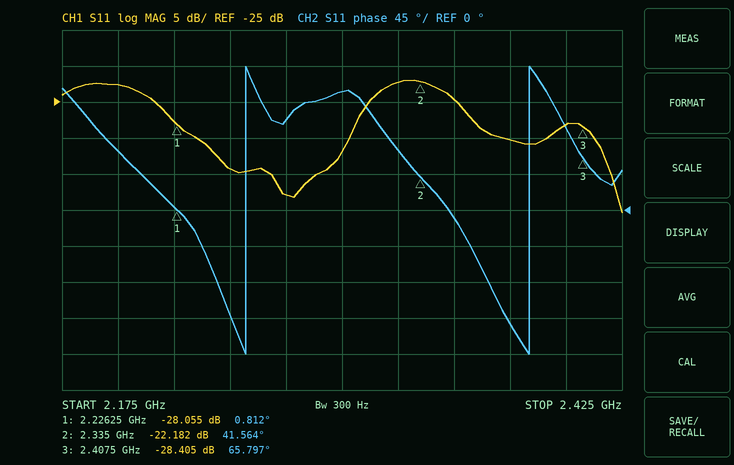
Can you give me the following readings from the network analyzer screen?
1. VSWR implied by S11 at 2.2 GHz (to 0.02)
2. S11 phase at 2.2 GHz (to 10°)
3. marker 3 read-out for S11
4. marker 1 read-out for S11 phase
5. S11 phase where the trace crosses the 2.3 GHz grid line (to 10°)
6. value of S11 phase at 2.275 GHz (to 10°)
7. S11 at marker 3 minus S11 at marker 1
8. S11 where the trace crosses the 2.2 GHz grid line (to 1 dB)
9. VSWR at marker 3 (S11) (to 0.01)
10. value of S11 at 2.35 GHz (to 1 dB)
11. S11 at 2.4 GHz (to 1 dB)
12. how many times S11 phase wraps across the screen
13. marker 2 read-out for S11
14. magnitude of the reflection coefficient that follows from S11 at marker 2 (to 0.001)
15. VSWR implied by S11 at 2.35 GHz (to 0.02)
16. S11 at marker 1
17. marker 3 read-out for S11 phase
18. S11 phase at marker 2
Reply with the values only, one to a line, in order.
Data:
1.16
70°
-28.405 dB
0.812°
150°
110°
-0.350 dB
-23 dB
1.08
-25 dB
-28 dB
2
-22.182 dB
0.078
1.12
-28.055 dB
65.797°
41.564°
